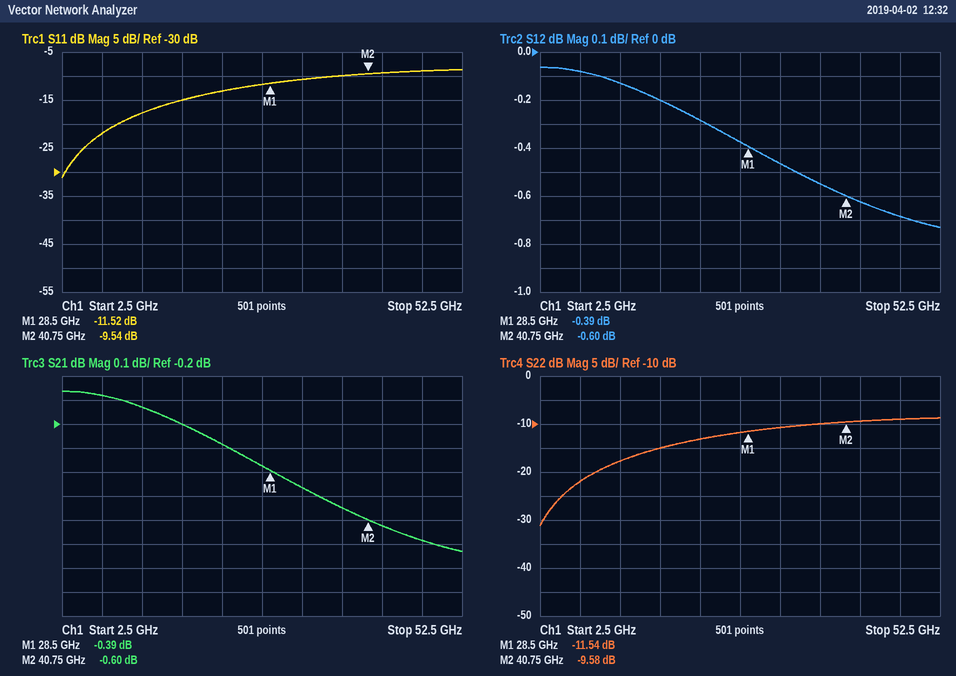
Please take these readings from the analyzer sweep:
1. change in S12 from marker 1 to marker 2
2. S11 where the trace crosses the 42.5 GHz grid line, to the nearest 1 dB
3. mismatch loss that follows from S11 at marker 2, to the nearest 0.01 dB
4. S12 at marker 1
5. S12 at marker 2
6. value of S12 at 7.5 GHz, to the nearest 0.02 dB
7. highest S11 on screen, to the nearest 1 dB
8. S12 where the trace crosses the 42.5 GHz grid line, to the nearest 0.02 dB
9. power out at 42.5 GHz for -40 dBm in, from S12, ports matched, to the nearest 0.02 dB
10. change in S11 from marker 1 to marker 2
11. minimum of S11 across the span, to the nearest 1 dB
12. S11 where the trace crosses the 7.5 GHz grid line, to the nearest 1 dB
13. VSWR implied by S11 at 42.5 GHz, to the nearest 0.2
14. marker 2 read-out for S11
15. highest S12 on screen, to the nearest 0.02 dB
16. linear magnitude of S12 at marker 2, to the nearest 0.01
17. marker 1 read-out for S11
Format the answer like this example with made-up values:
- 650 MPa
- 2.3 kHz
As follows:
- -0.21 dB
- -9 dB
- 0.51 dB
- -0.39 dB
- -0.60 dB
- -0.08 dB
- -9 dB
- -0.62 dB
- -40.62 dBm
- 1.98 dB
- -31 dB
- -22 dB
- 2.0
- -9.54 dB
- -0.06 dB
- 0.93
- -11.52 dB
